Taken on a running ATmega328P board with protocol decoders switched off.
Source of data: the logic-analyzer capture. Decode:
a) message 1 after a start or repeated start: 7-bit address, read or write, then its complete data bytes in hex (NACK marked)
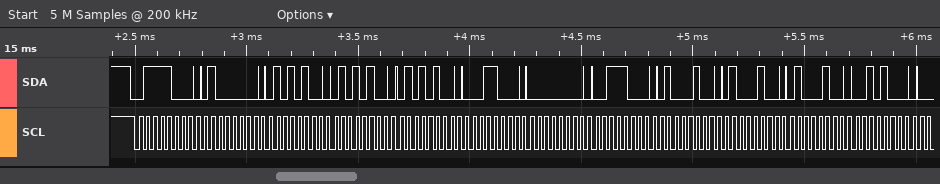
0x3C write: 40 54 54 54 18 00 38 44 44 44 28
